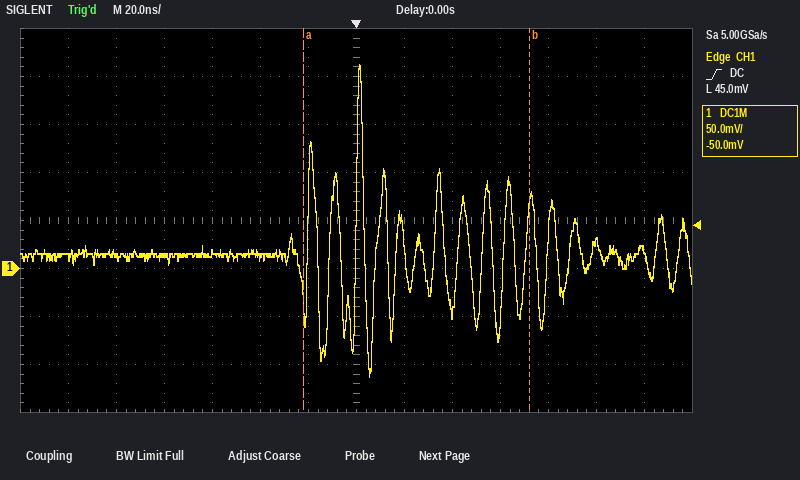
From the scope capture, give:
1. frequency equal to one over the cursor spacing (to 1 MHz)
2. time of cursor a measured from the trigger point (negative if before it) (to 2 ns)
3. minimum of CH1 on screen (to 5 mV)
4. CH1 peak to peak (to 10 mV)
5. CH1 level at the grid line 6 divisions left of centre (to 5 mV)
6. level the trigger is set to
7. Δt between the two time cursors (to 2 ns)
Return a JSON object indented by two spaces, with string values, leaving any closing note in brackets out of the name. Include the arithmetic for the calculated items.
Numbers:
{
  "frequency equal to one over the cursor spacing": "1 / 94 ns ≈ 11 MHz",
  "time of cursor a measured from the trigger point (negative if before it)": "-22 ns",
  "minimum of CH1 on screen": "-110 mV",
  "CH1 peak to peak": "320 mV",
  "CH1 level at the grid line 6 divisions left of centre": "10 mV",
  "level the trigger is set to": "45.0 mV",
  "Δt between the two time cursors": "94 ns"
}
